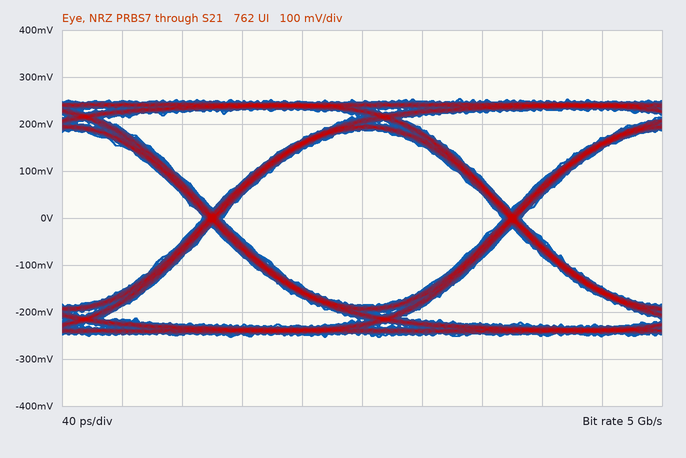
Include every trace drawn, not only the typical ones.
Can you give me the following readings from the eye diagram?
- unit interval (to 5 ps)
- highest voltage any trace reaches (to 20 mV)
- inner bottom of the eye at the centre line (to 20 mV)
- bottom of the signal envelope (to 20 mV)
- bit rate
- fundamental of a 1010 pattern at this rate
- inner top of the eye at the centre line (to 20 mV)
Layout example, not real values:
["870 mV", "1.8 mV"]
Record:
["200 ps", "260 mV", "-180 mV", "-260 mV", "5 Gb/s", "2.5 GHz", "180 mV"]
